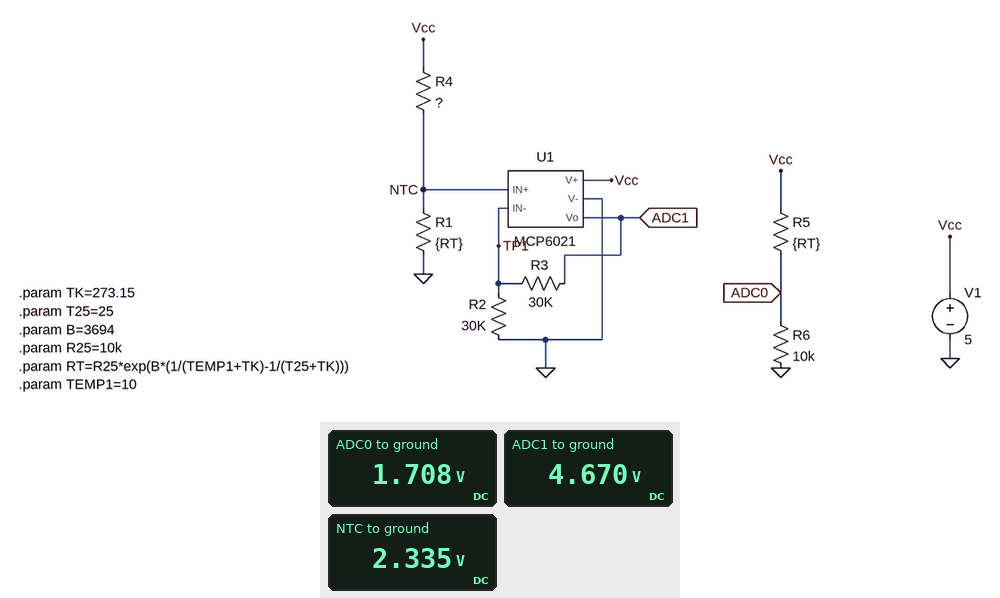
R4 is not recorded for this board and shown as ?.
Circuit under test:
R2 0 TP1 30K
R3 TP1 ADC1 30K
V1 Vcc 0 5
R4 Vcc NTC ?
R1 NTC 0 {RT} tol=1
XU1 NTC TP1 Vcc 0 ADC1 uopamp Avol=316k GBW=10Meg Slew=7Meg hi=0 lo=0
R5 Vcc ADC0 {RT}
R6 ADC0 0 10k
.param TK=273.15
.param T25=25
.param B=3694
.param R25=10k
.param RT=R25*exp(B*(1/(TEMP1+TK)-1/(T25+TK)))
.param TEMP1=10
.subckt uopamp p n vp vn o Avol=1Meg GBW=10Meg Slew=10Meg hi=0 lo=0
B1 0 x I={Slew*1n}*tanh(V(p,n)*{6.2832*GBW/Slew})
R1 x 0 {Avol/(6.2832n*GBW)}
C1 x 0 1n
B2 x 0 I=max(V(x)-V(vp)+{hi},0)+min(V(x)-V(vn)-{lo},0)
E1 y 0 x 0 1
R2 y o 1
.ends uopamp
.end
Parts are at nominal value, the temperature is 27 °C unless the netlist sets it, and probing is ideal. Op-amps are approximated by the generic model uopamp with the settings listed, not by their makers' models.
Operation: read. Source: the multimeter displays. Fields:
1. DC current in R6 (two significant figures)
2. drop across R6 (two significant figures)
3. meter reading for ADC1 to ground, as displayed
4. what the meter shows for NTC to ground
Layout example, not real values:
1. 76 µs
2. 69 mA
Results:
1. 170 µA
2. 1.7 V
3. 4.670 V
4. 2.335 V
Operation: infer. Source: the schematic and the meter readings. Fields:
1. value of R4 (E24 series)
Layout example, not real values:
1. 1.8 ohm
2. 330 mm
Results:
1. 22 kΩ
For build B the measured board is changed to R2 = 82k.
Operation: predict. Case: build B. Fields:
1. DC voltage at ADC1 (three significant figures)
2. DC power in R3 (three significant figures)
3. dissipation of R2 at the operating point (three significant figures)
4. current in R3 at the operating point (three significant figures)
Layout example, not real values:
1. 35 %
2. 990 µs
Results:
1. 3.19 V
2. 24.3 µW
3. 66.5 µW
4. 28.5 µA
